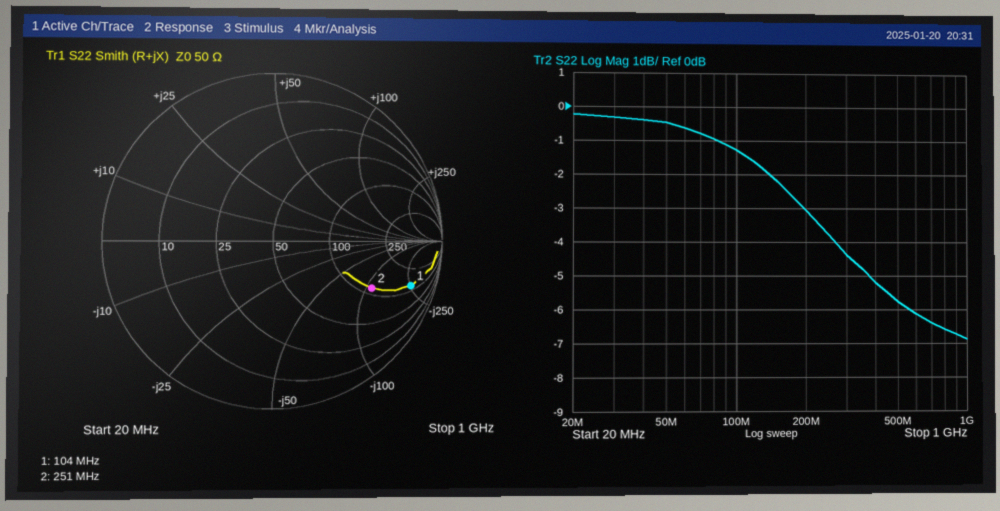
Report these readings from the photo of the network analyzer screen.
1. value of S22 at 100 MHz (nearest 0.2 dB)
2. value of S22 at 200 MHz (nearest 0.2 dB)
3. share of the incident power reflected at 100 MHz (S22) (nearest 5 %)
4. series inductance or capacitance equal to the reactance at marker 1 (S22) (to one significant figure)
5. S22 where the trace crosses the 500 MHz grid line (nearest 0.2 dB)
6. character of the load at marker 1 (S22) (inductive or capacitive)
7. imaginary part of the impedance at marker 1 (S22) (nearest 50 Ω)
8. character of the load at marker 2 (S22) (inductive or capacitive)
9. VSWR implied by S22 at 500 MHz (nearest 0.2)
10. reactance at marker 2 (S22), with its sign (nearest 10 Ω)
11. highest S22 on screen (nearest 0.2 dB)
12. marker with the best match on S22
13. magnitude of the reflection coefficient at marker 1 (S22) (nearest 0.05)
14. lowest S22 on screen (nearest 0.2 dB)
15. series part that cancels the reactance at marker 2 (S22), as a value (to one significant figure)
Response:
-1.2 dB
-3.0 dB
75 %
6 pF
-5.8 dB
capacitive
-250 Ω
capacitive
3.2
-110 Ω
-0.2 dB
marker 2
0.85
-6.8 dB
70 nH
